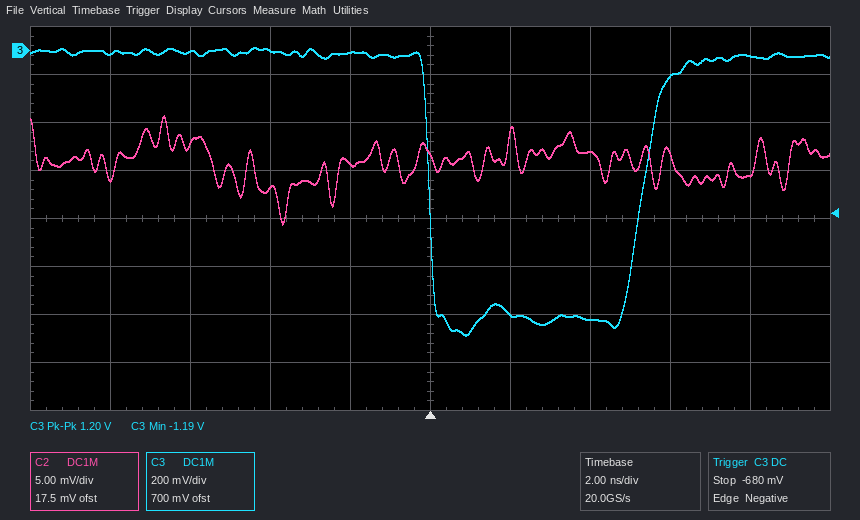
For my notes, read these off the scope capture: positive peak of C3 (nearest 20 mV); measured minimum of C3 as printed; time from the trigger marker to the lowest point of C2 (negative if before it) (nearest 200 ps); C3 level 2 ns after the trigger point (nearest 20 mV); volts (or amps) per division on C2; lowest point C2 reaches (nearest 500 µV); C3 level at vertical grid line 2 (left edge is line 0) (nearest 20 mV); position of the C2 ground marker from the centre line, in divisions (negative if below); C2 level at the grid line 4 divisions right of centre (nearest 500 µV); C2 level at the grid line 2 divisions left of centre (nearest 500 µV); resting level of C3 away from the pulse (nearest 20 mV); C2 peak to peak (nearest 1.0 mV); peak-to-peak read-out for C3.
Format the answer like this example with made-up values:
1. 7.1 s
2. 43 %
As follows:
1. 20 mV
2. -1.19 V
3. -3.6 ns
4. -1.10 V
5. 5 mV
6. -18.0 mV
7. 0 mV
8. +3.5 div
9. -12.5 mV
10. -14.5 mV
11. -20 mV
12. 11.0 mV
13. 1.20 V
